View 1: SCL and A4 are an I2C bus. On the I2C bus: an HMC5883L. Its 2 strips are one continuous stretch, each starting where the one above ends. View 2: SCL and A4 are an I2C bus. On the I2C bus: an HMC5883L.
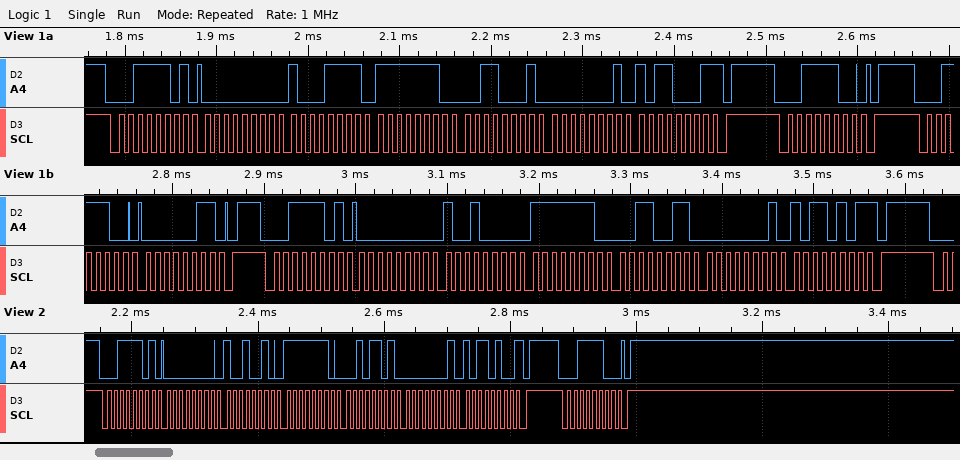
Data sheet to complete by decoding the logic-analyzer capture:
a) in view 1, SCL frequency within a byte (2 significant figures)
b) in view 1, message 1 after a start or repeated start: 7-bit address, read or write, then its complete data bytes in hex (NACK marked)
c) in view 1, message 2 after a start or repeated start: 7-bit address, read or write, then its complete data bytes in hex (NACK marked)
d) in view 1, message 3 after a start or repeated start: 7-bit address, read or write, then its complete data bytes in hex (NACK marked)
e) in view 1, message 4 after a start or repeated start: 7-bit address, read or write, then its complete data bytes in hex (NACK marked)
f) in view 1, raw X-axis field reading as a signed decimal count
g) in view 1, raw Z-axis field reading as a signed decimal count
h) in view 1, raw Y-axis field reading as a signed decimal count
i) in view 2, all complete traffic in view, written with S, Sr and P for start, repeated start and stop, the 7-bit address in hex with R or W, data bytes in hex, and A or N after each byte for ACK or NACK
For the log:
100 kHz
0x1E read: 00 8F FE 31 01 B1 NACK
0x1E write
0x1E write: 03
0x1E read: 00 90 FE 33 01 B5 NACK
144
-461
437
S 1ER A 00 A 92 A FE A 2D A 01 A B4 N P S 1EW A P
